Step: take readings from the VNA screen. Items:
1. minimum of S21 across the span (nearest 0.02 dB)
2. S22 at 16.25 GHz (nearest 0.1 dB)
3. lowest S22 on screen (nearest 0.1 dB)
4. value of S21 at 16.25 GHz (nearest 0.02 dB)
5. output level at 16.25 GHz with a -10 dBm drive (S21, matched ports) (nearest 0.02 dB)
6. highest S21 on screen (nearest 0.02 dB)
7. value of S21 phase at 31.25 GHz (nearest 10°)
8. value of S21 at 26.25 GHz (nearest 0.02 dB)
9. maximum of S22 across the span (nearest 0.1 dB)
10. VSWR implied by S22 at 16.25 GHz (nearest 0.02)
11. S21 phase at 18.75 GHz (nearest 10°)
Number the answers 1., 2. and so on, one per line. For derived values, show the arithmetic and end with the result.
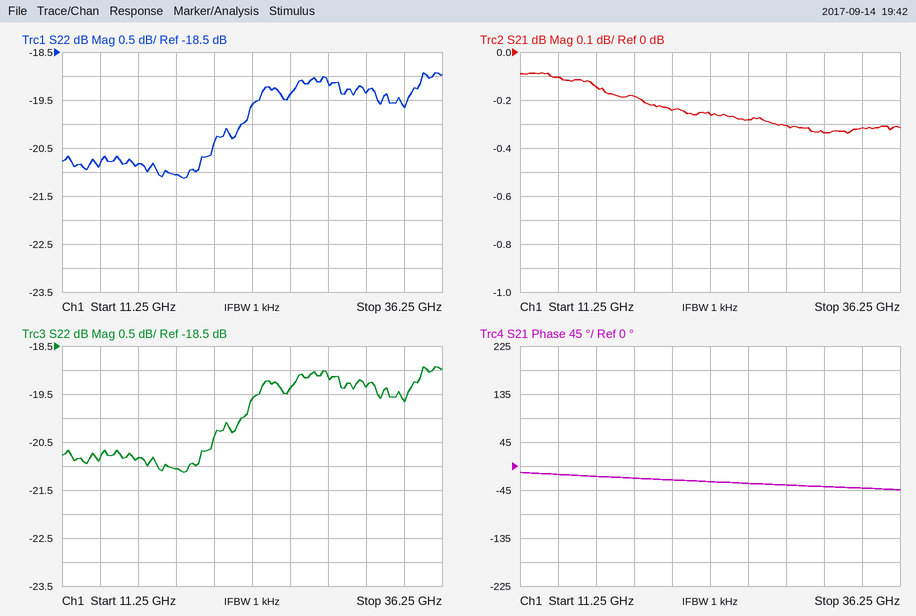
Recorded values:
1. -0.34 dB
2. -20.8 dB
3. -21.1 dB
4. -0.14 dB
5. -10 dBm + (-0.14 dB) = -10.14 dBm
6. -0.08 dB
7. -40°
8. -0.28 dB
9. -18.9 dB
10. |Γ| = 10^(-20.8/20) = 0.0912; VSWR = (1 + 0.0912)/(1 − 0.0912) ≈ 1.20
11. -20°
